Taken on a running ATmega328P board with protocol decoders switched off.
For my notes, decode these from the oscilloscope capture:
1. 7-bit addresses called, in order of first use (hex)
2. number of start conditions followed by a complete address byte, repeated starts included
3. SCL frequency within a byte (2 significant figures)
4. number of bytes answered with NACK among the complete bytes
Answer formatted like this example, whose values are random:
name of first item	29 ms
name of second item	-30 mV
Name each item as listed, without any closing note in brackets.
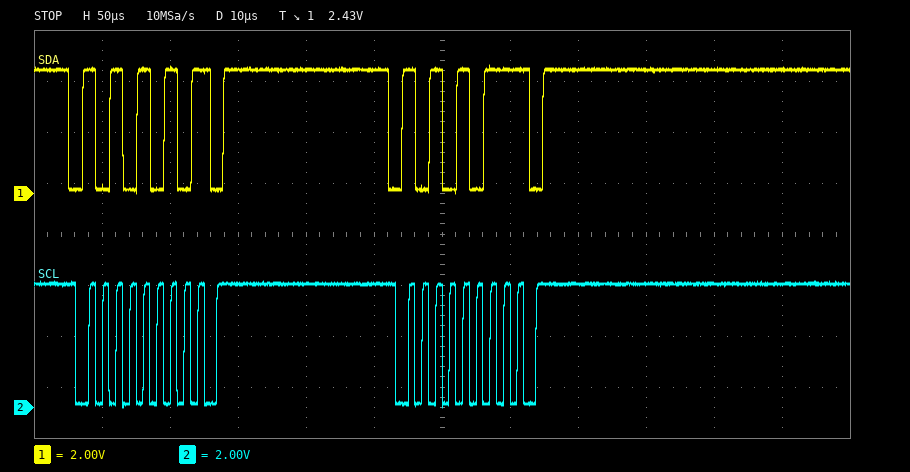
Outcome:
7-bit addresses called, in order of first use	0x55
number of start conditions followed by a complete address byte, repeated starts included	2
SCL frequency within a byte	100 kHz
number of bytes answered with NACK among the complete bytes	2
